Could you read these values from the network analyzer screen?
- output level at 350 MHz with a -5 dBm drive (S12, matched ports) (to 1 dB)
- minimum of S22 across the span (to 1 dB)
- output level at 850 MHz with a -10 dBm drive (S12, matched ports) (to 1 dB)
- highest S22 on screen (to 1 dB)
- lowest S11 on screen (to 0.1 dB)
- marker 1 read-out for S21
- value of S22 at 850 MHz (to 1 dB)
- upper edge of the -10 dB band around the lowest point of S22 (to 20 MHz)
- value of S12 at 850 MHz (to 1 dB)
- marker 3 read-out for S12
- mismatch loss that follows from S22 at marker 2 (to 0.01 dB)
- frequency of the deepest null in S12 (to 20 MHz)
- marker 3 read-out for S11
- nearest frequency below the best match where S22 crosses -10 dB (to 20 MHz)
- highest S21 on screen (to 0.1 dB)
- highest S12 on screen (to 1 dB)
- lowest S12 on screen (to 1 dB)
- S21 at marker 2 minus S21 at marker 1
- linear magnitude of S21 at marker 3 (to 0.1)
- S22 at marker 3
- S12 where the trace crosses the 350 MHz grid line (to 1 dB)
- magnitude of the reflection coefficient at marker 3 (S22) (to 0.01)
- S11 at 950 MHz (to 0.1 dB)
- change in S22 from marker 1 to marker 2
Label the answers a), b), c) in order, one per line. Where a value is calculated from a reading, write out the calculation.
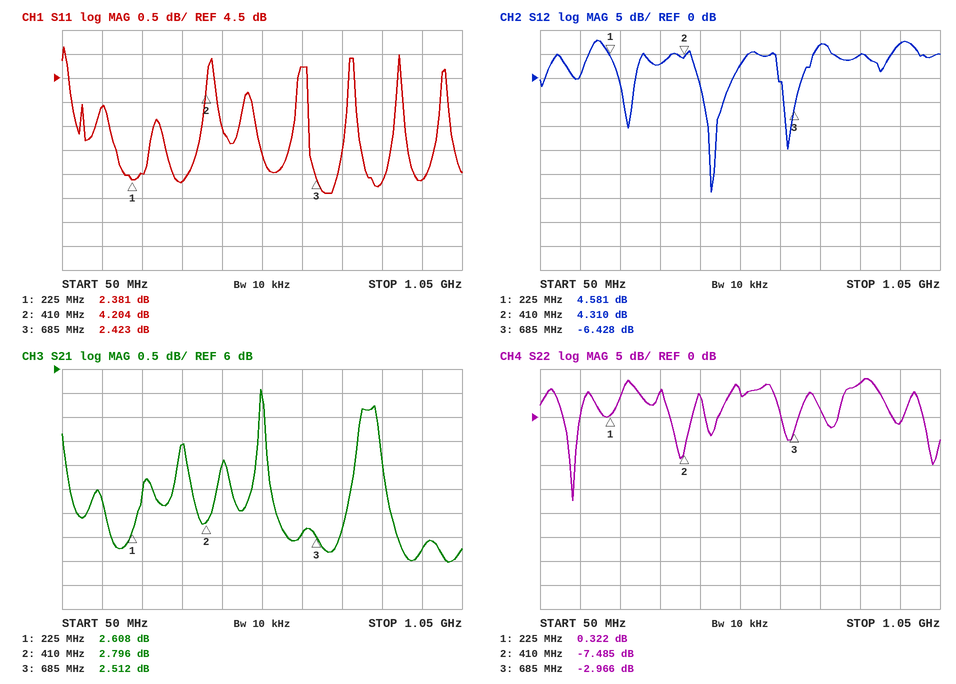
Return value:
a) -5 dBm + (3 dB) = -2 dBm
b) -17 dB
c) -10 dBm + (5 dB) = -5 dBm
d) 8 dB
e) 2.1 dB
f) 2.608 dB
g) 7 dB
h) 140 MHz
i) 5 dB
j) -6.428 dB
k) −10 log10(1 − 10^(-7.485/10)) ≈ 0.85 dB
l) 480 MHz
m) 2.423 dB
n) 120 MHz
o) 5.6 dB
p) 8 dB
q) -24 dB
r) 2.796 − (2.608) = 0.188 dB
s) 10^(2.512/20) ≈ 1.3
t) -2.966 dB
u) 3 dB
v) 10^(-2.966/20) ≈ 0.71
w) 2.4 dB
x) -7.485 − (0.322) = -7.807 dB
